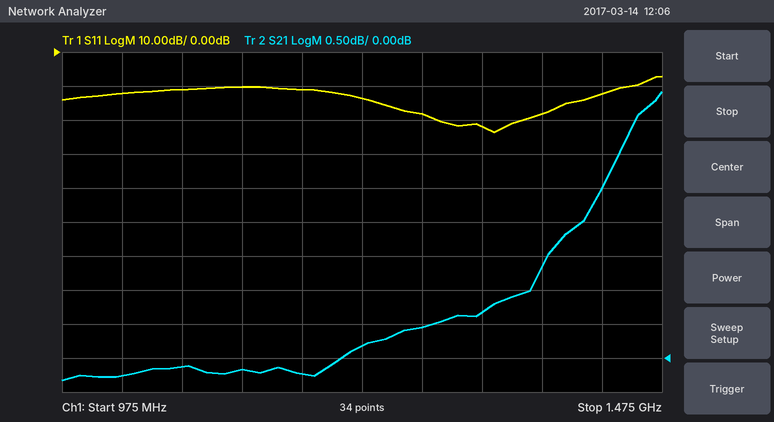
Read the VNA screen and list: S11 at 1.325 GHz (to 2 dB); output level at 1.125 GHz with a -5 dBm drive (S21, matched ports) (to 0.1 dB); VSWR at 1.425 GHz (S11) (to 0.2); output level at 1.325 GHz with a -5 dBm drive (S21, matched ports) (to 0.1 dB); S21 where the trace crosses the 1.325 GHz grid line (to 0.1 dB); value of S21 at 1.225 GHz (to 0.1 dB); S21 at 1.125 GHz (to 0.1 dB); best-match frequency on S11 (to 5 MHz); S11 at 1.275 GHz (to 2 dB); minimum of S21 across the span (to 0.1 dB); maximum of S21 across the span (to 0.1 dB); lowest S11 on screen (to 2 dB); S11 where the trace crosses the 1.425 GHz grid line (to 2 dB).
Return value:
-22 dB
-5.2 dBm
1.6
-4.3 dBm
0.7 dB
0.2 dB
-0.2 dB
1.335 GHz
-18 dB
-0.3 dB
3.9 dB
-24 dB
-12 dB
